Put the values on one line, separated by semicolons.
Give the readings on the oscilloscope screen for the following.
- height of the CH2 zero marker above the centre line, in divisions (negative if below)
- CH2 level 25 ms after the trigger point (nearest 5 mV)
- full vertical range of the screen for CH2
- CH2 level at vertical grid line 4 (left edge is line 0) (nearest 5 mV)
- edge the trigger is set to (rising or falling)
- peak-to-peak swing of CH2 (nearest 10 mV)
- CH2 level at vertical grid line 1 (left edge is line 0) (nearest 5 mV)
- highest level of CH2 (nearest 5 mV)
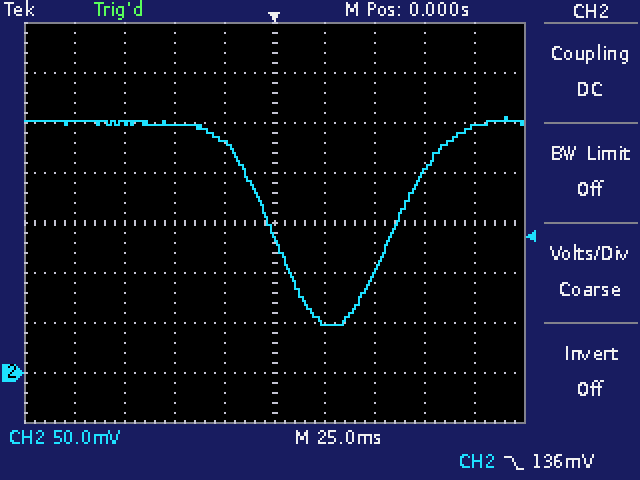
-3.0 div; 50 mV; 400 mV; 230 mV; falling; 210 mV; 250 mV; 255 mV
